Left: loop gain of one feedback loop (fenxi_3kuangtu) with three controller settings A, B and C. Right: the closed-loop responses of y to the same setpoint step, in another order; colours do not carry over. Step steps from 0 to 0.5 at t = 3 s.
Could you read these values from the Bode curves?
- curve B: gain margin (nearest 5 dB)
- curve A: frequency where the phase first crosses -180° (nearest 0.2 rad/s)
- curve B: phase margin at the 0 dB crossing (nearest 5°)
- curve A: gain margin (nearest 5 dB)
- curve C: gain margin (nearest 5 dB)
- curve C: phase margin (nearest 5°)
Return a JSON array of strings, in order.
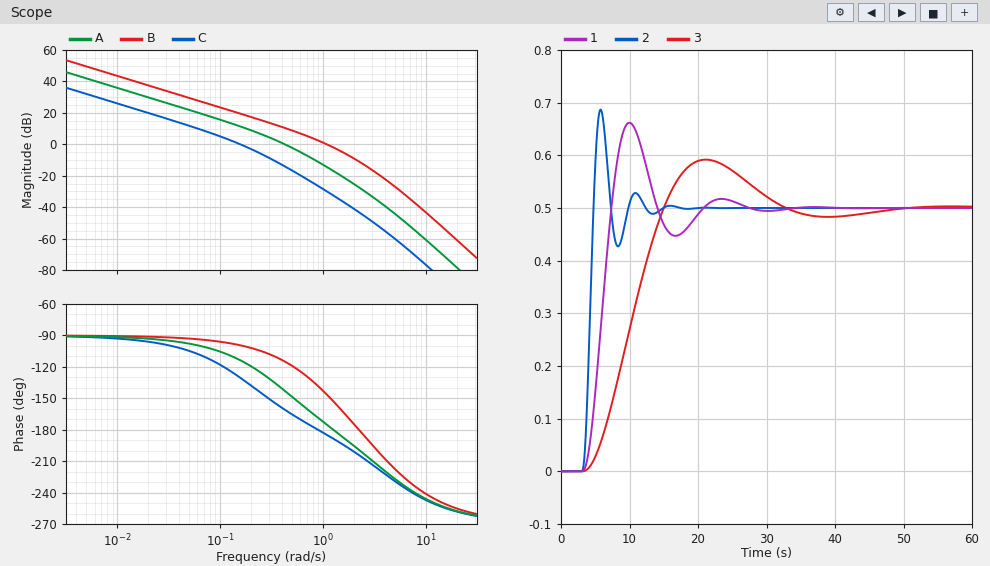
["10 dB", "1.2 rad/s", "35°", "15 dB", "25 dB", "50°"]
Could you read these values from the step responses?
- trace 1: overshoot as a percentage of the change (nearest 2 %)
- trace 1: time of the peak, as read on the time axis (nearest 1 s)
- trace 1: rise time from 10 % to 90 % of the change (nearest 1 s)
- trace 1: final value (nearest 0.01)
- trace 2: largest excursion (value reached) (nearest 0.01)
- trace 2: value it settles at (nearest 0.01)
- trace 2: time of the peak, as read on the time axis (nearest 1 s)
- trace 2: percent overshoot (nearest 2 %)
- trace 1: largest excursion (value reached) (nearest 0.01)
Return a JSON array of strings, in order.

["32 %", "10 s", "3 s", "0.50", "0.69", "0.50", "6 s", "38 %", "0.66"]
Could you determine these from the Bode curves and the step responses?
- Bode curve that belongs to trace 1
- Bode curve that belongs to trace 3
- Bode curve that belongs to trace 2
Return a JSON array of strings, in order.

["A", "C", "B"]
